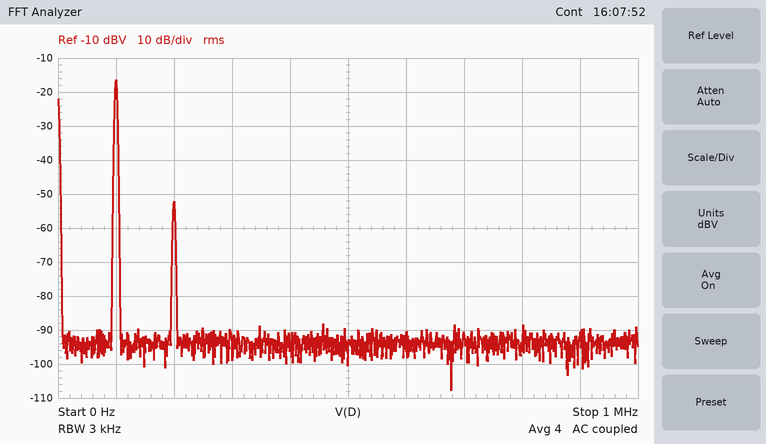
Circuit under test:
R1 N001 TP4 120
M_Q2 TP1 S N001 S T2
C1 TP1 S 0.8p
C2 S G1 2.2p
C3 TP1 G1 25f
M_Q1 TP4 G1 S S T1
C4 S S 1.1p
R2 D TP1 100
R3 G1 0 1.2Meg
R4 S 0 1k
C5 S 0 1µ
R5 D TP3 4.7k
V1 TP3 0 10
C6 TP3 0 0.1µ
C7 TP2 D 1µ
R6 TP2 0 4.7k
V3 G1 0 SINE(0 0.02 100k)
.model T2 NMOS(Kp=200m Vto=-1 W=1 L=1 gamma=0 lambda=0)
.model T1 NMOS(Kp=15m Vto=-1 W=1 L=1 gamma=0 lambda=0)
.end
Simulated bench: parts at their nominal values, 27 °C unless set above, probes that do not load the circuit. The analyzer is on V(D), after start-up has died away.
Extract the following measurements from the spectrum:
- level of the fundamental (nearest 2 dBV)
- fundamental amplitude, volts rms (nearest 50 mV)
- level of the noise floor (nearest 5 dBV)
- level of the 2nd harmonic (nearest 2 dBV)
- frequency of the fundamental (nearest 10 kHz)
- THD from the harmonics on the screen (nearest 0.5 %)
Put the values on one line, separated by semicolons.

-16 dBV; 150 mV; -95 dBV; -52 dBV; 100 kHz; 1.5 %
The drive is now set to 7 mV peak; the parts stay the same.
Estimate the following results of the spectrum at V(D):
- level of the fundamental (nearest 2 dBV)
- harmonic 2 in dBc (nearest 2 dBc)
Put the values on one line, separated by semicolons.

-26 dBV; -44 dBc
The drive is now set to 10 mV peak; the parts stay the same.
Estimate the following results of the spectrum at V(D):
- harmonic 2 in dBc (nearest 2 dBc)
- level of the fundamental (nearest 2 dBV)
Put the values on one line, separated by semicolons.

-42 dBc; -22 dBV
